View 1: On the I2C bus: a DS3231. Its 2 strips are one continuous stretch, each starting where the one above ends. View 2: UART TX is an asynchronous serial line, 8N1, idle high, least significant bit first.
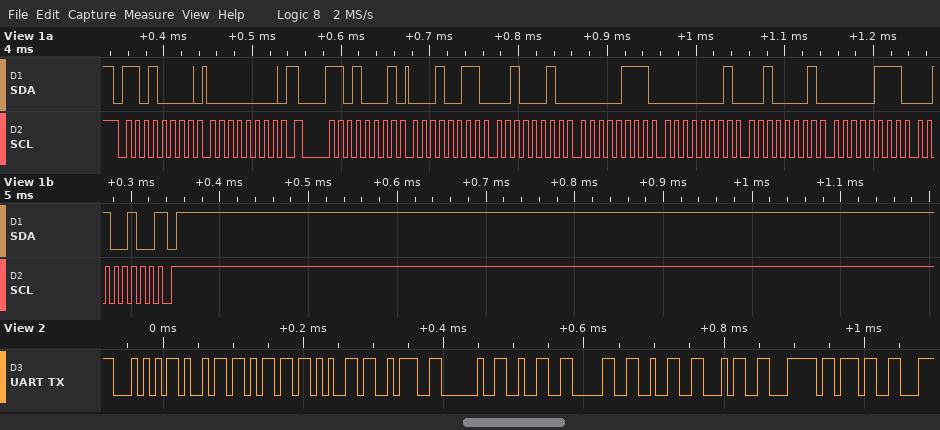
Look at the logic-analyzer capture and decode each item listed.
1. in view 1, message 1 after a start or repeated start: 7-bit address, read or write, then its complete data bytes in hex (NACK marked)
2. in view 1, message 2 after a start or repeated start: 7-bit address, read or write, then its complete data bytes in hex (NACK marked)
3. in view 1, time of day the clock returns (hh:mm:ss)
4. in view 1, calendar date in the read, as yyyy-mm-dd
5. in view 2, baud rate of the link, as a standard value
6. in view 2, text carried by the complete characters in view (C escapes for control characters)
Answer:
0x68 write: 00
0x68 read: 13 22 07 01 21 07 24 NACK
07:22:13
2024-07-21
115200 baud
"Time: 2024|7"
